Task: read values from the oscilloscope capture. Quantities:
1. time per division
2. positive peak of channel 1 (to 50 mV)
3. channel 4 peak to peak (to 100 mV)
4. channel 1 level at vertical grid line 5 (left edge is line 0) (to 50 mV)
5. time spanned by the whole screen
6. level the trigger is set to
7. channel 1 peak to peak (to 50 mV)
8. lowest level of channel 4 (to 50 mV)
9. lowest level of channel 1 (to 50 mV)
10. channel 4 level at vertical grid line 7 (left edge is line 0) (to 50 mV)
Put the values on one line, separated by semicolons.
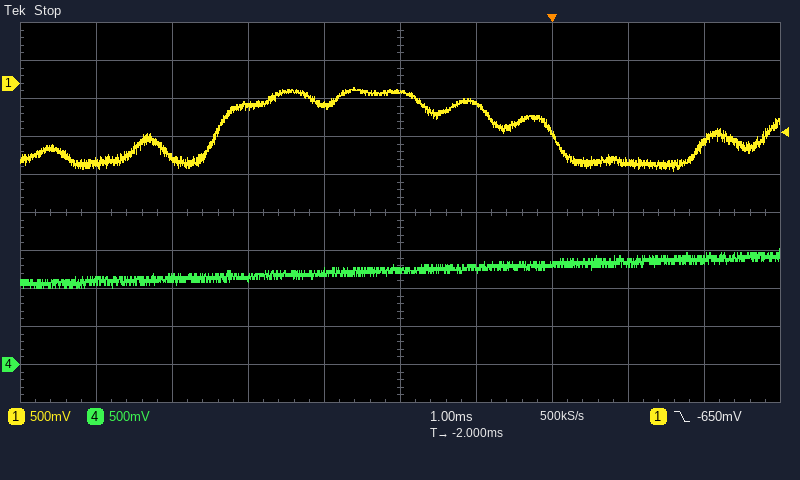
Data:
1 ms; -50 mV; 500 mV; -100 mV; 10 ms; -650 mV; 1.10 V; 1.00 V; -1.15 V; 1.30 V
